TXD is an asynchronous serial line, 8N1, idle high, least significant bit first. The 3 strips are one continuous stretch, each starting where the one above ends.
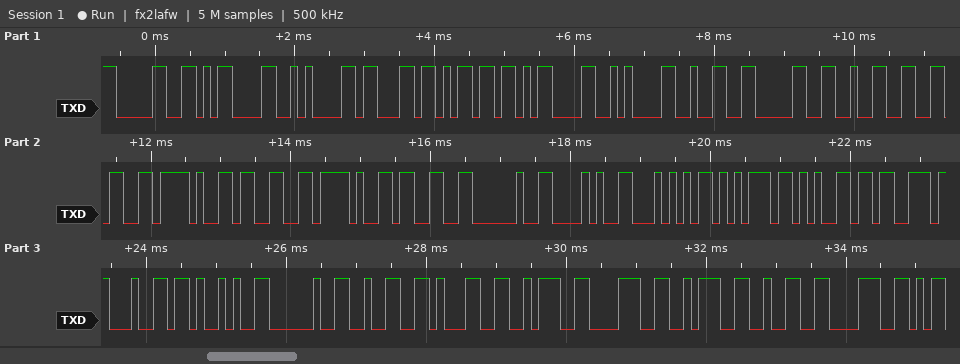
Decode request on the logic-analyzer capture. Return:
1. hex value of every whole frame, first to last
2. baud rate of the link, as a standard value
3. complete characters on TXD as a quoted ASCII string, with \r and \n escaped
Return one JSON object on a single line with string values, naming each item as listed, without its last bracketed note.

{"hex value of every whole frame, first to last": "30 0D 0A 63 6D 0D 0A 32 30 32 36 2F 33 2F 33 20 28 54 75 65 73 64 29 20 32 31 3A 38 3A 32 38", "baud rate of the link, as a standard value": "9600 baud", "complete characters on TXD as a quoted ASCII string, with \\r and \\n escaped": "\"0\\r\\ncm\\r\\n2026/3/3 (Tuesd) 21:8:28\""}
